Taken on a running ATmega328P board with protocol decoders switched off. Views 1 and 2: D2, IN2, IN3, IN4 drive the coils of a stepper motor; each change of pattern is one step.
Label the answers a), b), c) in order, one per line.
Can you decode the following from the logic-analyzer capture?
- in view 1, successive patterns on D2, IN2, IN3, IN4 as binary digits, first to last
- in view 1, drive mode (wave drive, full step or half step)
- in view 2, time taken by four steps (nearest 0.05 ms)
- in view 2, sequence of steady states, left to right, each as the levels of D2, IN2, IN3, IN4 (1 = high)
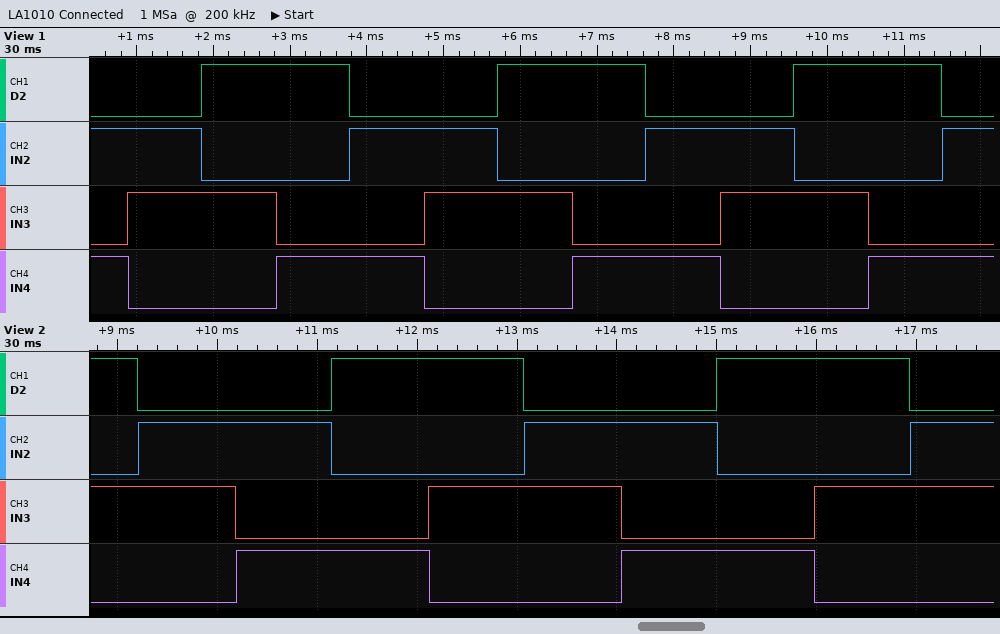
a) 0101 0110 1010 1001 0101 0110 1010 1001 0101 0110 1010 1001 0101
b) full step
c) 3.85 ms
d) 1010 0110 0101 1001 1010 0110 0101 1001 1010 0110
